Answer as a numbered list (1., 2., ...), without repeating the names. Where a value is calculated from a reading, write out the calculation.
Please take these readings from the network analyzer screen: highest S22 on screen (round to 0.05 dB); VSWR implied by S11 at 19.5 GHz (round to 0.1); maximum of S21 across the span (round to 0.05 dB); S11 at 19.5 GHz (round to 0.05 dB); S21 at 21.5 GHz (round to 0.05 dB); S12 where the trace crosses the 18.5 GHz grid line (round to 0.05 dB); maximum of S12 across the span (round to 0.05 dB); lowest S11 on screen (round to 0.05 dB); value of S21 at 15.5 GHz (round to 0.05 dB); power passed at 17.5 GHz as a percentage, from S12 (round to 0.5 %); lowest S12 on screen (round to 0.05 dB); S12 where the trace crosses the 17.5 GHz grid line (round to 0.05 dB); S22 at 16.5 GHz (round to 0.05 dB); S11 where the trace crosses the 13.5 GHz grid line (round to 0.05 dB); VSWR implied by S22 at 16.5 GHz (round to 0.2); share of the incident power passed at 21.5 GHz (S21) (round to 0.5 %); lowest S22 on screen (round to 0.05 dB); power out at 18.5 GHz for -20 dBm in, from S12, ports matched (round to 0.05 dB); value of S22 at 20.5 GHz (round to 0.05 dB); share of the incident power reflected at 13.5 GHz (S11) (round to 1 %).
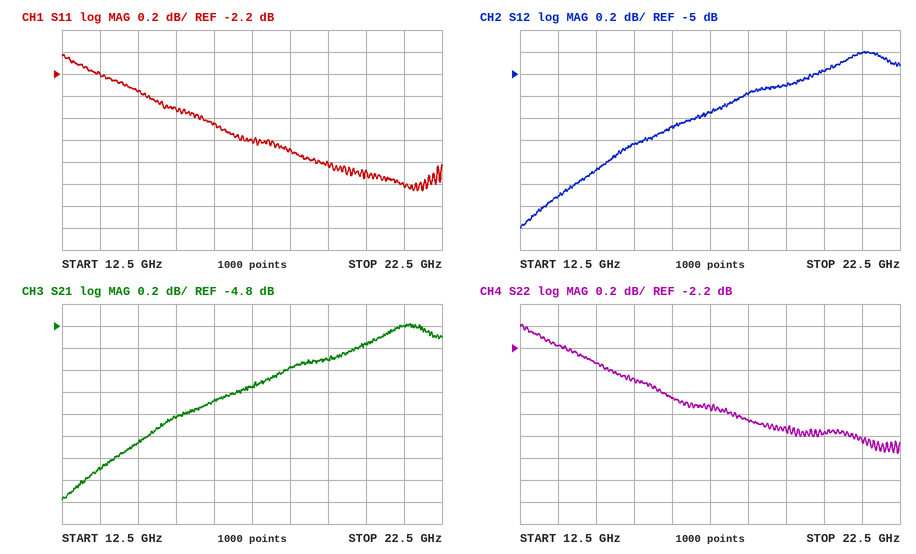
1. -2.00 dB
2. |Γ| = 10^(-3/20) = 0.7079; VSWR = (1 + 0.7079)/(1 − 0.7079) ≈ 5.8
3. -4.80 dB
4. -3.00 dB
5. -4.80 dB
6. -5.20 dB
7. -4.80 dB
8. -3.25 dB
9. -5.65 dB
10. 10^(-5.35/10) ≈ 29.2 %, so 29.0 % to the nearest 0.5 %
11. -6.40 dB
12. -5.35 dB
13. -2.65 dB
14. -2.20 dB
15. |Γ| = 10^(-2.65/20) = 0.7371; VSWR = (1 + 0.7371)/(1 − 0.7371) ≈ 6.6
16. 10^(-4.8/10) ≈ 33.1 %, so 33.0 % to the nearest 0.5 %
17. -3.15 dB
18. -20 dBm + (-5.20 dB) = -25.20 dBm
19. -2.95 dB
20. 10^(-2.2/10) ≈ 60 %
